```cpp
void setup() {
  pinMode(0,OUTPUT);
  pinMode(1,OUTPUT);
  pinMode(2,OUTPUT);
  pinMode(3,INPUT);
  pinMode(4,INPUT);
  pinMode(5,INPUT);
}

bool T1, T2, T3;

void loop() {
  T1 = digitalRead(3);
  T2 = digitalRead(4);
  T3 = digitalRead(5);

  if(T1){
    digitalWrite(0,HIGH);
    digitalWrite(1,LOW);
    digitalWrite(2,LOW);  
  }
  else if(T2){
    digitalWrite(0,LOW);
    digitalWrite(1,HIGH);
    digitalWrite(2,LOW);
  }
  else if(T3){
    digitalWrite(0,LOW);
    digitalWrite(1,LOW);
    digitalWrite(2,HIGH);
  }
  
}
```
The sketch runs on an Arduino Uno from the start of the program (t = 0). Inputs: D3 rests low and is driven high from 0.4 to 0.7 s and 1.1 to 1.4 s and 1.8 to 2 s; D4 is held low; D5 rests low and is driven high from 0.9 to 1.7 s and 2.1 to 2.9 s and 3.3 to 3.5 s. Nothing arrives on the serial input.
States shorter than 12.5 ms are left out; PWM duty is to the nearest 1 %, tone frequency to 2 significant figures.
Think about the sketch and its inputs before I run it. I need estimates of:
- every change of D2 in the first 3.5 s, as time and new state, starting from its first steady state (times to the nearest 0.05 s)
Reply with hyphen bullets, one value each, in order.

- 0 s low; 0.9 s high; 1.1 s low; 1.4 s high; 1.8 s low; 2.1 s high
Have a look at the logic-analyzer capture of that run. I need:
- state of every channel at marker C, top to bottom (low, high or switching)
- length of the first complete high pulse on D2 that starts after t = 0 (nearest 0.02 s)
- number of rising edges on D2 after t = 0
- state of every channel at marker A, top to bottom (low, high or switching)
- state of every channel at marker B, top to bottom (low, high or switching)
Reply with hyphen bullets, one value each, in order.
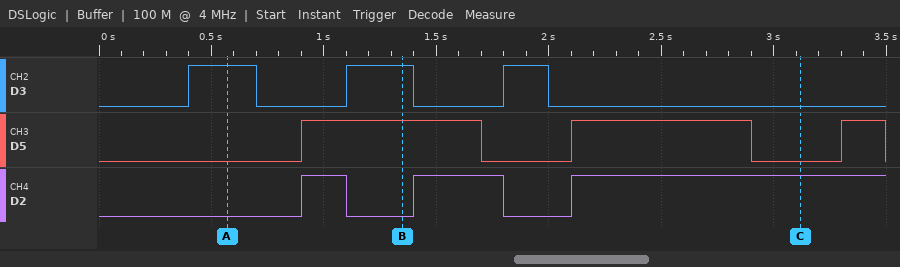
- D3 low, D5 low, D2 high
- 0.20 s
- 3
- D3 high, D5 low, D2 low
- D3 high, D5 high, D2 low
